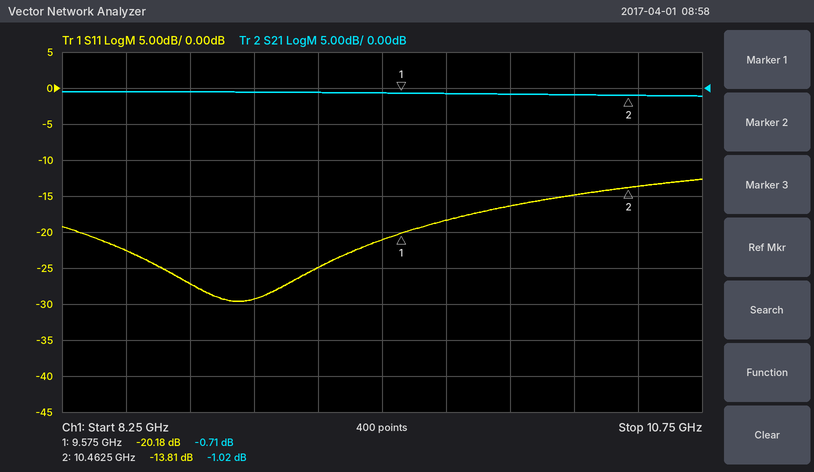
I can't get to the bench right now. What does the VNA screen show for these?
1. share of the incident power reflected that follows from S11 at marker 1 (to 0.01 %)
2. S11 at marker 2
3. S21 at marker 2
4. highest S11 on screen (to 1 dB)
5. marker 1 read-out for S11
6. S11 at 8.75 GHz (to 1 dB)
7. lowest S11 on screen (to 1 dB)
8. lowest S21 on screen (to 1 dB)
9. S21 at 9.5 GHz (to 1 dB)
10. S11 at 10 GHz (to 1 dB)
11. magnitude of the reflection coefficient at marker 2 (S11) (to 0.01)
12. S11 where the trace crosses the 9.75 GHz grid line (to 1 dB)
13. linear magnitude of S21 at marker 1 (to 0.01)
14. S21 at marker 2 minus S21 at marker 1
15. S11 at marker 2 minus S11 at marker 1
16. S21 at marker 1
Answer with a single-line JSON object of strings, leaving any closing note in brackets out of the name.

{"share of the incident power reflected that follows from S11 at marker 1": "0.96 %", "S11 at marker 2": "-13.81 dB", "S21 at marker 2": "-1.02 dB", "highest S11 on screen": "-13 dB", "marker 1 read-out for S11": "-20.18 dB", "S11 at 8.75 GHz": "-27 dB", "lowest S11 on screen": "-30 dB", "lowest S21 on screen": "-1 dB", "S21 at 9.5 GHz": "-1 dB", "S11 at 10 GHz": "-16 dB", "magnitude of the reflection coefficient at marker 2 (S11)": "0.20", "S11 where the trace crosses the 9.75 GHz grid line": "-18 dB", "linear magnitude of S21 at marker 1": "0.92", "S21 at marker 2 minus S21 at marker 1": "-0.31 dB", "S11 at marker 2 minus S11 at marker 1": "6.37 dB", "S21 at marker 1": "-0.71 dB"}
